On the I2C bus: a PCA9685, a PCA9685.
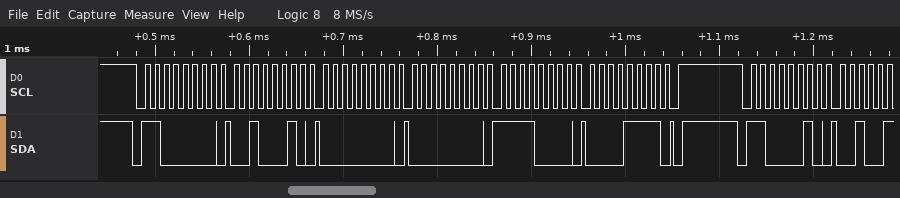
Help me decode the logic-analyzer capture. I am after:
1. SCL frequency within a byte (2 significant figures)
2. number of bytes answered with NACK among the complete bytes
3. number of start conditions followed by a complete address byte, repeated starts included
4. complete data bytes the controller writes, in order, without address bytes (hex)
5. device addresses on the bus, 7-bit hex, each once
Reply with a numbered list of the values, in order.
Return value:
1. 100 kHz
2. 0
3. 2
4. 22 00 00 F0 0F
5. 0x60 0x61
